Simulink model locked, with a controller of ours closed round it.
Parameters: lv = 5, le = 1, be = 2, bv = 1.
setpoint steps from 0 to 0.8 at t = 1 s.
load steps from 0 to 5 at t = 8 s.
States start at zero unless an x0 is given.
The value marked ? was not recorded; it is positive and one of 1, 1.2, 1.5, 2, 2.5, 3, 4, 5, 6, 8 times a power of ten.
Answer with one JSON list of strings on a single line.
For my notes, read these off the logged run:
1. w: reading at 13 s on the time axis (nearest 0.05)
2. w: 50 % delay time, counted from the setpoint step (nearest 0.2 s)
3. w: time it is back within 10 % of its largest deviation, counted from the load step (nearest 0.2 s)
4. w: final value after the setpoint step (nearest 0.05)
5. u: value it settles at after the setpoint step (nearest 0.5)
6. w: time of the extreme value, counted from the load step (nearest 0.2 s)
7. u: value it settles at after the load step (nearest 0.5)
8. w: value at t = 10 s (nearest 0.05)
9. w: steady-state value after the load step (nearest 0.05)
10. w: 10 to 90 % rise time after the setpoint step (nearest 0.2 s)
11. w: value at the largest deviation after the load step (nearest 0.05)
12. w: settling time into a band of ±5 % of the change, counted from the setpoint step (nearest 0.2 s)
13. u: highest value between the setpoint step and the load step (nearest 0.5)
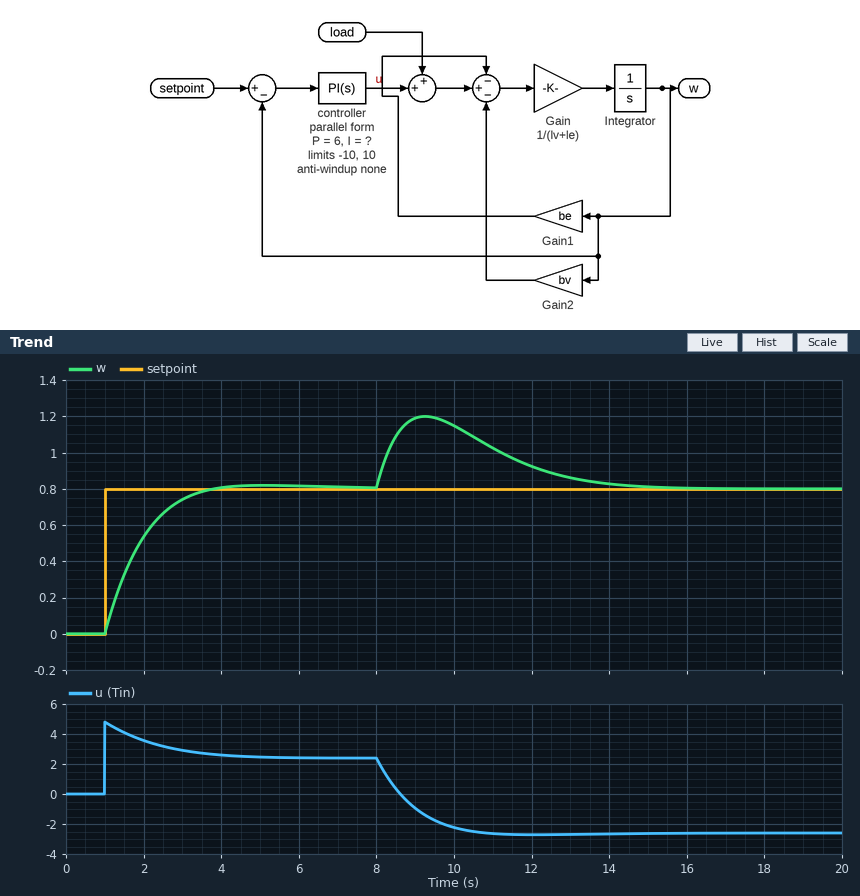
["0.85", "0.6 s", "5.6 s", "0.80", "2.5", "1.2 s", "-2.5", "1.15", "0.80", "1.8 s", "1.20", "2.2 s", "5.0"]
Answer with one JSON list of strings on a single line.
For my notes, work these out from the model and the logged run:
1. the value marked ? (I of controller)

["4"]
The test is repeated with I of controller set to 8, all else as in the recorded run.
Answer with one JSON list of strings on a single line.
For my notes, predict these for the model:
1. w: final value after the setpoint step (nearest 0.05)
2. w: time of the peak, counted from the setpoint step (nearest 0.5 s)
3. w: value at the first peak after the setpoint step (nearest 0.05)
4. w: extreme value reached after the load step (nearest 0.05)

["0.80", "2.5 s", "0.90", "1.15"]
